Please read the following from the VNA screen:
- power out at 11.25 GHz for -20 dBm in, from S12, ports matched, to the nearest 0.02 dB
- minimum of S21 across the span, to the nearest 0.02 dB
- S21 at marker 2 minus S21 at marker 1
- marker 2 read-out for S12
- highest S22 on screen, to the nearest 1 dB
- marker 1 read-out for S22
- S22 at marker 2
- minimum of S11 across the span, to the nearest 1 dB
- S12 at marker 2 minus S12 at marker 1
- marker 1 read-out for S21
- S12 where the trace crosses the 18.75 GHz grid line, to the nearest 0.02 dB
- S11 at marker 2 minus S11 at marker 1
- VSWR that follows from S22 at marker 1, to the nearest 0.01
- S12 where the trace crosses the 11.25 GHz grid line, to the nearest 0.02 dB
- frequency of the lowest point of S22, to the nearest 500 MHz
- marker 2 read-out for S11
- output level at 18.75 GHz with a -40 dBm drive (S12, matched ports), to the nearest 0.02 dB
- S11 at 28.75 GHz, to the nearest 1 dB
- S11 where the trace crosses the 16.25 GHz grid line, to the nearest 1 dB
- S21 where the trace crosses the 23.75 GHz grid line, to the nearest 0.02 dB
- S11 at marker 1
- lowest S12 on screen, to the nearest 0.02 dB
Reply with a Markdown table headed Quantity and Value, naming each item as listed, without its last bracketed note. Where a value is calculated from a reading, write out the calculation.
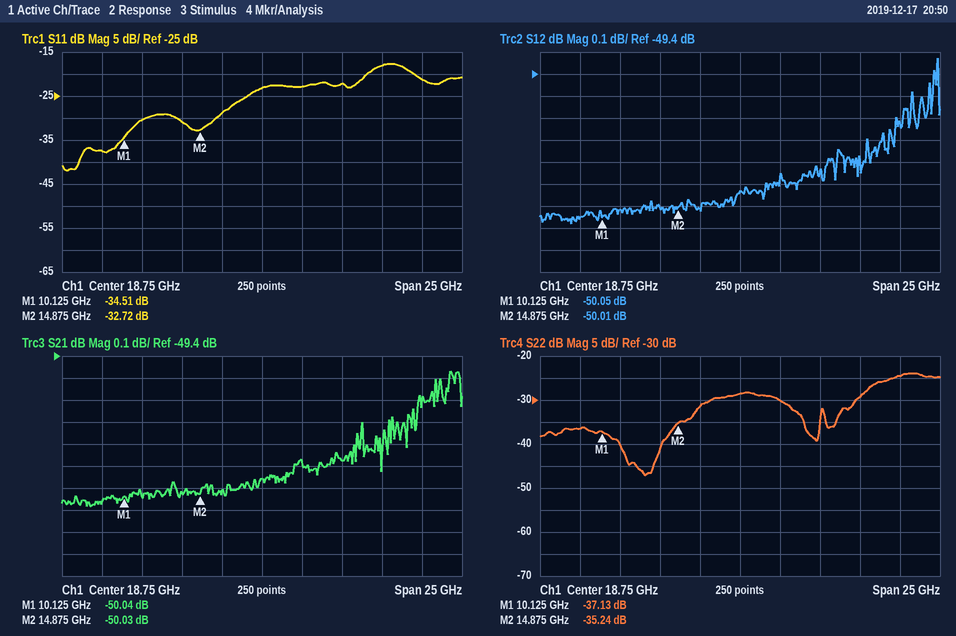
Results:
| Quantity | Value |
|---|---|
| power out at 11.25 GHz for -20 dBm in, from S12, ports matched, to the nearest 0.02 dB | -20 dBm + (-50.02 dB) = -70.02 dBm |
| minimum of S21 across the span, to the nearest 0.02 dB | -50.08 dB |
| S21 at marker 2 minus S21 at marker 1 | -50.03 − (-50.04) = 0.01 dB |
| marker 2 read-out for S12 | -50.01 dB |
| highest S22 on screen, to the nearest 1 dB | -24 dB |
| marker 1 read-out for S22 | -37.13 dB |
| S22 at marker 2 | -35.24 dB |
| minimum of S11 across the span, to the nearest 1 dB | -42 dB |
| S12 at marker 2 minus S12 at marker 1 | -50.01 − (-50.05) = 0.04 dB |
| marker 1 read-out for S21 | -50.04 dB |
| S12 where the trace crosses the 18.75 GHz grid line, to the nearest 0.02 dB | -49.94 dB |
| S11 at marker 2 minus S11 at marker 1 | -32.72 − (-34.51) = 1.79 dB |
| VSWR that follows from S22 at marker 1, to the nearest 0.01 | (1 + 0.0139)/(1 − 0.0139) ≈ 1.03 |
| S12 where the trace crosses the 11.25 GHz grid line, to the nearest 0.02 dB | -50.02 dB |
| frequency of the lowest point of S22, to the nearest 500 MHz | 13.0 GHz |
| marker 2 read-out for S11 | -32.72 dB |
| output level at 18.75 GHz with a -40 dBm drive (S12, matched ports), to the nearest 0.02 dB | -40 dBm + (-49.94 dB) = -89.94 dBm |
| S11 at 28.75 GHz, to the nearest 1 dB | -21 dB |
| S11 where the trace crosses the 16.25 GHz grid line, to the nearest 1 dB | -29 dB |
| S21 where the trace crosses the 23.75 GHz grid line, to the nearest 0.02 dB | -49.88 dB |
| S11 at marker 1 | -34.51 dB |
| lowest S12 on screen, to the nearest 0.02 dB | -50.08 dB |
